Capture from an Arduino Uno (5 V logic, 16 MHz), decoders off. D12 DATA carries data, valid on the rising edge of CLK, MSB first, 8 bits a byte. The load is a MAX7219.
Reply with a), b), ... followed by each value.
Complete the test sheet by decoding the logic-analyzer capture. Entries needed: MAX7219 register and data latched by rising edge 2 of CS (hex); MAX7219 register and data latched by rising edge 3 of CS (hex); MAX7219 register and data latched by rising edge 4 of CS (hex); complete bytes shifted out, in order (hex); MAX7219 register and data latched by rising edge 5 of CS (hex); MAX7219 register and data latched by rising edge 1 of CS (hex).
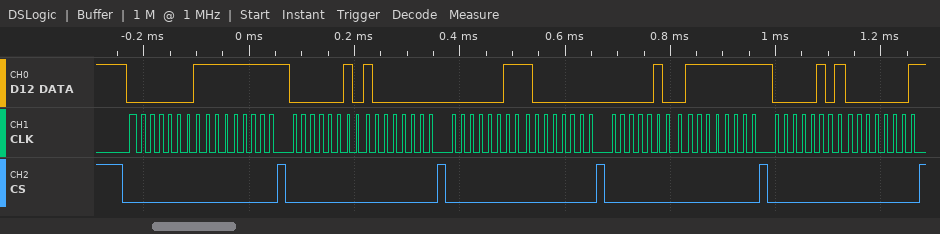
a) register 0x2, data 0x80
b) register 0x3, data 0x80
c) register 0x4, data 0xFF
d) 01 FF 02 80 03 80 04 FF 05 01
e) register 0x5, data 0x01
f) register 0x1, data 0xFF
